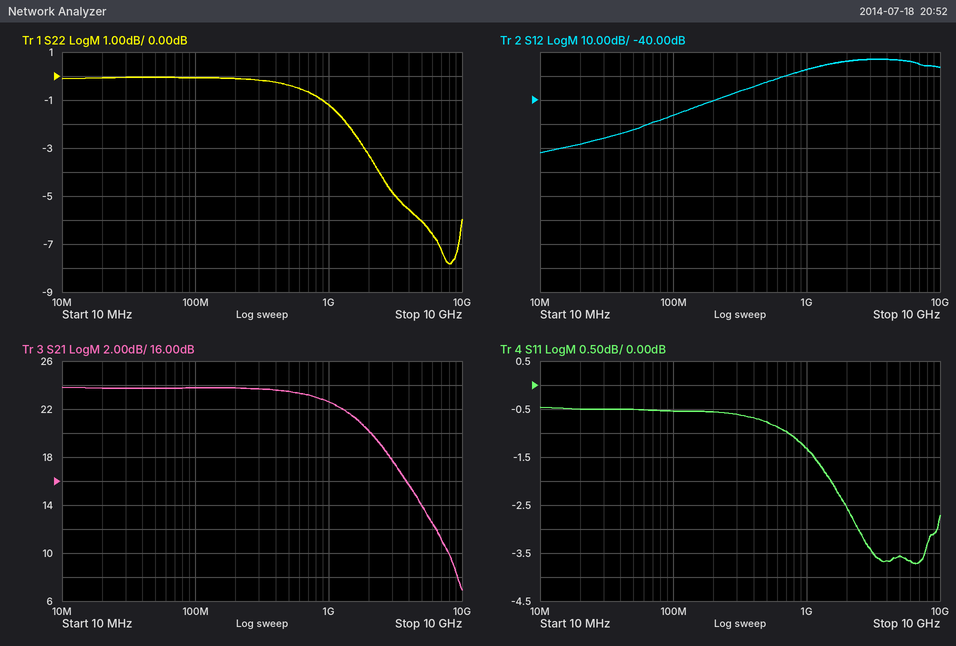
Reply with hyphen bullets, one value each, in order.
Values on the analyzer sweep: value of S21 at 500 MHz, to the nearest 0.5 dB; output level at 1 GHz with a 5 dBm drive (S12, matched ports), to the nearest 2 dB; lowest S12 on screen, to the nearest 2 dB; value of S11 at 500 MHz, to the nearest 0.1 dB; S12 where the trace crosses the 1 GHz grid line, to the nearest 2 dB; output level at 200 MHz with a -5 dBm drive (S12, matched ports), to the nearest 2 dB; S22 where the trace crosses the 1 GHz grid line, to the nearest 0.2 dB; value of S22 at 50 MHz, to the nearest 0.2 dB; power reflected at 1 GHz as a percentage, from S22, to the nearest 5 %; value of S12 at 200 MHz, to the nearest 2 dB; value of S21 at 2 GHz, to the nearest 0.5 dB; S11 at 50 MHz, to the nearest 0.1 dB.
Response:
- 23.5 dB
- -22 dBm
- -62 dB
- -0.8 dB
- -28 dB
- -46 dBm
- -1.2 dB
- 0.0 dB
- 75 %
- -40 dB
- 20.0 dB
- -0.5 dB
